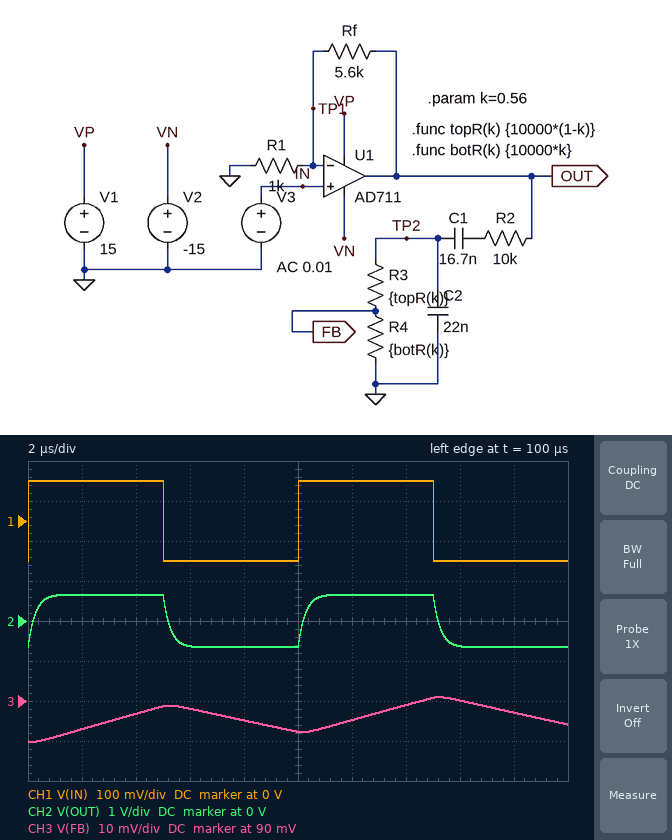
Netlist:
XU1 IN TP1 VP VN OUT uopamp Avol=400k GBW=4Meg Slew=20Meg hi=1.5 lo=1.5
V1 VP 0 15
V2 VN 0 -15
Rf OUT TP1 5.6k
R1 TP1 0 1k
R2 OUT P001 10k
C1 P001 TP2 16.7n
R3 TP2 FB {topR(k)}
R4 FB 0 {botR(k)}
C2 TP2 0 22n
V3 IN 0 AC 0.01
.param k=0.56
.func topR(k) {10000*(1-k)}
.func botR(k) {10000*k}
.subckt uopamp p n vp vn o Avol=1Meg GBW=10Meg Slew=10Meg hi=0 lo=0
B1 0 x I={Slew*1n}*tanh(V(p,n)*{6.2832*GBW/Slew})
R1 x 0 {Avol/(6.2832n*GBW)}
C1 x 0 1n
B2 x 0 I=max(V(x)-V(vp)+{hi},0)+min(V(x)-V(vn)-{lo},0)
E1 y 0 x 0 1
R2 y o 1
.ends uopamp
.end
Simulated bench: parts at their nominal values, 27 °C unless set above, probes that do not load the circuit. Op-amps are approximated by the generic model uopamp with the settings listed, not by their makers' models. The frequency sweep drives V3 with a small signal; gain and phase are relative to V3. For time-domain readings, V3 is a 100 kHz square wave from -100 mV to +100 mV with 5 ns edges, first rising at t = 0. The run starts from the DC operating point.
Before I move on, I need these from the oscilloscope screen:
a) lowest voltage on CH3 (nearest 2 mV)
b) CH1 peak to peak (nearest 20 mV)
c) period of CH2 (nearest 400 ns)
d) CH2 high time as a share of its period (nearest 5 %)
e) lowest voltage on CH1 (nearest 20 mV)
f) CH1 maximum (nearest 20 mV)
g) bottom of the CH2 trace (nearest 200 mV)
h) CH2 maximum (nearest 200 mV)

80 mV
200 mV
10.0 µs
50 %
-100 mV
100 mV
-600 mV
600 mV
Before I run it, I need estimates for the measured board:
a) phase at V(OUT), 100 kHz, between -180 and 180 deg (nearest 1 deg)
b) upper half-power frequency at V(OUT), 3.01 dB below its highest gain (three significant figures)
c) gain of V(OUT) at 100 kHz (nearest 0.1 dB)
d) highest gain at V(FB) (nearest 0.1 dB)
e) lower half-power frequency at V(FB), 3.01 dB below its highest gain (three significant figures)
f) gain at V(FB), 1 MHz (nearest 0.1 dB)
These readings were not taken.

-9 deg
606 kHz
16.3 dB
0.9 dB
259 Hz
-57.2 dB
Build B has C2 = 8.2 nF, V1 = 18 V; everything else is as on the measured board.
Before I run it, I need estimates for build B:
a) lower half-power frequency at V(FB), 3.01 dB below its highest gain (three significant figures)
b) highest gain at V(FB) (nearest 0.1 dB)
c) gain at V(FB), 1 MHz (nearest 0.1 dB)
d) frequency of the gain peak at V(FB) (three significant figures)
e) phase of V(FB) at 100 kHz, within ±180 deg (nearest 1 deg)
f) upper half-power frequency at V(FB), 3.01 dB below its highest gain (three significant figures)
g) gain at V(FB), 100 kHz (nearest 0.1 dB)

356 Hz
3.4 dB
-48.6 dB
1.36 kHz
-97 deg
5.19 kHz
-23.0 dB
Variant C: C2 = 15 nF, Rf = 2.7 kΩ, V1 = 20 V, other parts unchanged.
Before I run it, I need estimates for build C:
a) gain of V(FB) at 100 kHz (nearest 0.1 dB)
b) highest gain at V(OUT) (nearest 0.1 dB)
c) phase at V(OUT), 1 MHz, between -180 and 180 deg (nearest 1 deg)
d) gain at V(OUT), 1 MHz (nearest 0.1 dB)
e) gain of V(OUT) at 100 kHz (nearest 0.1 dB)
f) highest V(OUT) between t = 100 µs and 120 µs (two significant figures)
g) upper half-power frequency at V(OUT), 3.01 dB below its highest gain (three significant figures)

-33.2 dB
11.4 dB
-43 deg
8.7 dB
11.3 dB
370 mV
1.08 MHz
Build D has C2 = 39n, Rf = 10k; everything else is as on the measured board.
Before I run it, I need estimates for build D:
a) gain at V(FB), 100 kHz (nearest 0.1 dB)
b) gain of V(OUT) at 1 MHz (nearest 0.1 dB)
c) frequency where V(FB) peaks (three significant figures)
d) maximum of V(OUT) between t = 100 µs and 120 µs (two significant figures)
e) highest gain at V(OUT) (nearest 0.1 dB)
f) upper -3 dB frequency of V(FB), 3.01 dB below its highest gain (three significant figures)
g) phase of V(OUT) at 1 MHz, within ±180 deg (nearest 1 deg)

-32.3 dB
11.5 dB
624 Hz
1.1 V
20.8 dB
1.97 kHz
-70 deg
